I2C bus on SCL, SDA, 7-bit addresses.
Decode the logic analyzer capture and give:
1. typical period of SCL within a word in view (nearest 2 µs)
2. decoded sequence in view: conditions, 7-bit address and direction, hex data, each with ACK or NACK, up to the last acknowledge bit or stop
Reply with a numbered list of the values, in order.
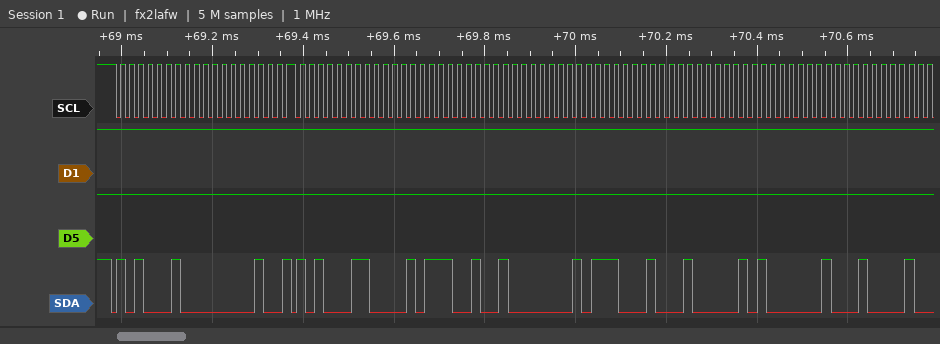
1. 20 µs
2. start, address 51 write ACK, 02 ACK, repeated start, address 51 read ACK, 17 ACK, 48 ACK, 17 ACK, 22 ACK, 14 ACK, 11 ACK
